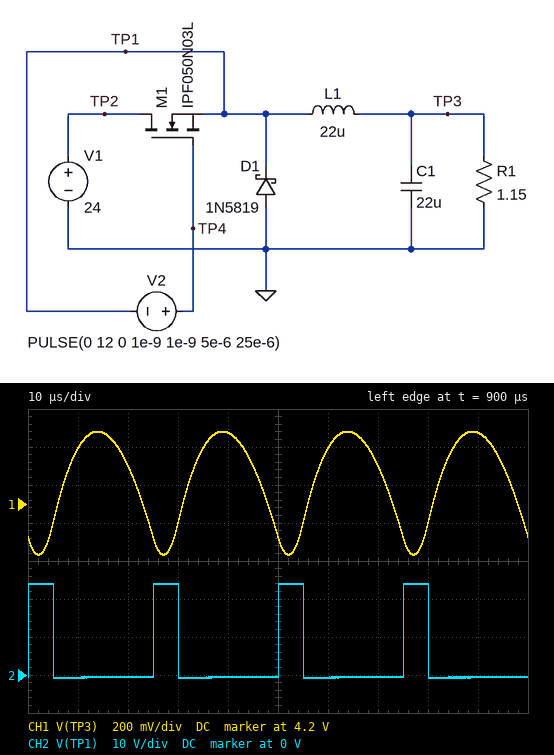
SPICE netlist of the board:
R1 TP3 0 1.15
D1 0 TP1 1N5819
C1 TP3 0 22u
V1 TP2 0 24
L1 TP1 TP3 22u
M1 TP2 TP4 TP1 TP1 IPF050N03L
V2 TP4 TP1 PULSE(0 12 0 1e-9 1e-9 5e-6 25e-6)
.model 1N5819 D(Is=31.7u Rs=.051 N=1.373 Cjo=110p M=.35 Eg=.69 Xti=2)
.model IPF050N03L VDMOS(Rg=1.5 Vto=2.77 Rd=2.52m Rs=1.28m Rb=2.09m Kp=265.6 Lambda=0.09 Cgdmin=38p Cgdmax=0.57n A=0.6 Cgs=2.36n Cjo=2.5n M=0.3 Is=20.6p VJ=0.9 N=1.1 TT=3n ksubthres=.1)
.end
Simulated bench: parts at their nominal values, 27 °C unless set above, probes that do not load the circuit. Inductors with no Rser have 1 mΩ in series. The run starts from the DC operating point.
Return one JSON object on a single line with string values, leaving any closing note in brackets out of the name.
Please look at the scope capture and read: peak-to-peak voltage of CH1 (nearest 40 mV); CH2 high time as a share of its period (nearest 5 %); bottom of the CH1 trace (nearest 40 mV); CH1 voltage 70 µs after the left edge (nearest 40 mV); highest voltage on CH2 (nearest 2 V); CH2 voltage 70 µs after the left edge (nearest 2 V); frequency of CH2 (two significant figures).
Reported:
{"peak-to-peak voltage of CH1": "640 mV", "CH2 high time as a share of its period": "20 %", "bottom of the CH1 trace": "3.92 V", "CH1 voltage 70 µs after the left edge": "4.40 V", "highest voltage on CH2": "24 V", "CH2 voltage 70 µs after the left edge": "0 V", "frequency of CH2": "40 kHz"}
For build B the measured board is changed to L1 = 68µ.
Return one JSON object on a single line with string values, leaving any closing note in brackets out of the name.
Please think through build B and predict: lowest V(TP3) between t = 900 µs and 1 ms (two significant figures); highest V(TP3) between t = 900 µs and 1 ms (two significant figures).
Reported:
{"lowest V(TP3) between t = 900 µs and 1 ms": "4.2 V", "highest V(TP3) between t = 900 µs and 1 ms": "4.4 V"}
